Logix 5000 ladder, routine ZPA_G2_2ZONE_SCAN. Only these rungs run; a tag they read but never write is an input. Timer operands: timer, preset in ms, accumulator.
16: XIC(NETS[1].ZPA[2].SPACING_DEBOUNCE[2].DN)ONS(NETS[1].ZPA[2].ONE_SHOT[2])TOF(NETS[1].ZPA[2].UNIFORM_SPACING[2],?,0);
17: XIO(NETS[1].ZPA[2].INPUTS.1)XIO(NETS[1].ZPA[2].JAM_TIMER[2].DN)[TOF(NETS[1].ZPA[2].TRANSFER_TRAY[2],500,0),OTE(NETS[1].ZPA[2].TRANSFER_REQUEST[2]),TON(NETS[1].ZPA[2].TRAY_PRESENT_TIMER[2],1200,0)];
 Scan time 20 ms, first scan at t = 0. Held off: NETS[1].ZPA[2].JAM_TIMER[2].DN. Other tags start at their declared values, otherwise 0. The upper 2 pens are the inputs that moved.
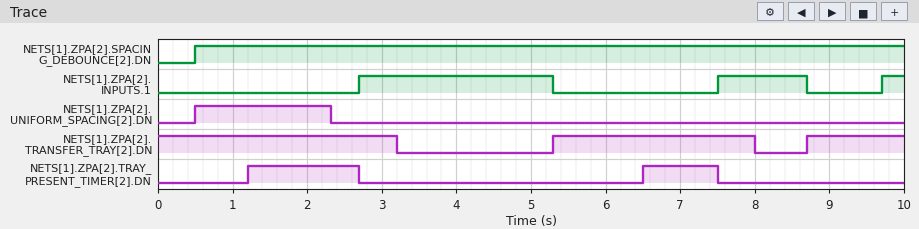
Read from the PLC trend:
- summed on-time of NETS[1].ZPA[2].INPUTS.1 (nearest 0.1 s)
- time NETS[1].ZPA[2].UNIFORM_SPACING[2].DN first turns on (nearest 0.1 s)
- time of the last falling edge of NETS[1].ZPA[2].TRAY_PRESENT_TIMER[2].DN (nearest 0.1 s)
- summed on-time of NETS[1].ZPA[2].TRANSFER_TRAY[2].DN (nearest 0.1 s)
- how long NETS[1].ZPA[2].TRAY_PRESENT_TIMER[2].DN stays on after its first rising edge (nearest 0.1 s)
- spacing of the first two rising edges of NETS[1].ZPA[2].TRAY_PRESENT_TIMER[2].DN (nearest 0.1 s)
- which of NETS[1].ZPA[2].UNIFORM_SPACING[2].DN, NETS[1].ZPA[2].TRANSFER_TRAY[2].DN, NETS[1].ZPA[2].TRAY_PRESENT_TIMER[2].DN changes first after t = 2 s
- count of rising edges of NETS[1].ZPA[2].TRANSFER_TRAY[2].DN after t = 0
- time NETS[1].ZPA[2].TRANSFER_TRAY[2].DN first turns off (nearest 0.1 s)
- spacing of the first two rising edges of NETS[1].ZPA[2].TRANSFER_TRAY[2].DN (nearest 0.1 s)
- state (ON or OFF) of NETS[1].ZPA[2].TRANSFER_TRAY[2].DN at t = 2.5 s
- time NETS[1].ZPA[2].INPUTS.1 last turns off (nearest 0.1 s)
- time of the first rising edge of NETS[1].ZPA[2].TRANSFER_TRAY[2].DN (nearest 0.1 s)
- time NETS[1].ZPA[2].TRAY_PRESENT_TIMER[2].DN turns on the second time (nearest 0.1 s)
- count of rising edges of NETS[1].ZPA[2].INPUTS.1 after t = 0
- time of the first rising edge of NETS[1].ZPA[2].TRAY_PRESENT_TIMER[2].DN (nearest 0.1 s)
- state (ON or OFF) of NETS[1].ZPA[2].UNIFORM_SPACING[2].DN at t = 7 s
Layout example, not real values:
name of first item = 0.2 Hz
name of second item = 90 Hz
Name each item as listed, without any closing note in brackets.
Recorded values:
summed on-time of NETS[1].ZPA[2].INPUTS.1 = 4.1 s
time NETS[1].ZPA[2].UNIFORM_SPACING[2].DN first turns on = 0.5 s
time of the last falling edge of NETS[1].ZPA[2].TRAY_PRESENT_TIMER[2].DN = 7.5 s
summed on-time of NETS[1].ZPA[2].TRANSFER_TRAY[2].DN = 7.2 s
how long NETS[1].ZPA[2].TRAY_PRESENT_TIMER[2].DN stays on after its first rising edge = 1.5 s
spacing of the first two rising edges of NETS[1].ZPA[2].TRAY_PRESENT_TIMER[2].DN = 5.3 s
which of NETS[1].ZPA[2].UNIFORM_SPACING[2].DN, NETS[1].ZPA[2].TRANSFER_TRAY[2].DN, NETS[1].ZPA[2].TRAY_PRESENT_TIMER[2].DN changes first after t = 2 s = NETS[1].ZPA[2].UNIFORM_SPACING[2].DN
count of rising edges of NETS[1].ZPA[2].TRANSFER_TRAY[2].DN after t = 0 = 2
time NETS[1].ZPA[2].TRANSFER_TRAY[2].DN first turns off = 3.2 s
spacing of the first two rising edges of NETS[1].ZPA[2].TRANSFER_TRAY[2].DN = 3.4 s
state (ON or OFF) of NETS[1].ZPA[2].TRANSFER_TRAY[2].DN at t = 2.5 s = ON
time NETS[1].ZPA[2].INPUTS.1 last turns off = 8.7 s
time of the first rising edge of NETS[1].ZPA[2].TRANSFER_TRAY[2].DN = 5.3 s
time NETS[1].ZPA[2].TRAY_PRESENT_TIMER[2].DN turns on the second time = 6.5 s
count of rising edges of NETS[1].ZPA[2].INPUTS.1 after t = 0 = 3
time of the first rising edge of NETS[1].ZPA[2].TRAY_PRESENT_TIMER[2].DN = 1.2 s
state (ON or OFF) of NETS[1].ZPA[2].UNIFORM_SPACING[2].DN at t = 7 s = OFF
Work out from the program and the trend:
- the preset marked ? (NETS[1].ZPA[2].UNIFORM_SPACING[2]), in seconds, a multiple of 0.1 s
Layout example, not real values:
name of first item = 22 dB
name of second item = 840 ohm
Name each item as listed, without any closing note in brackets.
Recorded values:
the preset marked ? (NETS[1].ZPA[2].UNIFORM_SPACING[2]), in seconds, a multiple of 0.1 s = 1.8 s
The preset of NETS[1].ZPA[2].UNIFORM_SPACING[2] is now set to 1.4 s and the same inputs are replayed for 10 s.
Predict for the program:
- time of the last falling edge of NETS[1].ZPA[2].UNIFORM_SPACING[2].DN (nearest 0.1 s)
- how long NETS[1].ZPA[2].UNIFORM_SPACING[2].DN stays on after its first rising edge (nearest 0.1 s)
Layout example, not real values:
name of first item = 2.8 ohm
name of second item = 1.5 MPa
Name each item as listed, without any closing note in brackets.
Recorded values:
time of the last falling edge of NETS[1].ZPA[2].UNIFORM_SPACING[2].DN = 1.9 s
how long NETS[1].ZPA[2].UNIFORM_SPACING[2].DN stays on after its first rising edge = 1.4 s
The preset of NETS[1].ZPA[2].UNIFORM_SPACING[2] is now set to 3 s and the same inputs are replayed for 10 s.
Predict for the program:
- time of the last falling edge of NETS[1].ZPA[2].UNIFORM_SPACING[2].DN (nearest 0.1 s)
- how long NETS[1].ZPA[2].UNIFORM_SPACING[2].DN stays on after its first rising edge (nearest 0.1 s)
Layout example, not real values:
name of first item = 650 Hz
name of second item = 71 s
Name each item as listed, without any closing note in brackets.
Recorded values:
time of the last falling edge of NETS[1].ZPA[2].UNIFORM_SPACING[2].DN = 3.5 s
how long NETS[1].ZPA[2].UNIFORM_SPACING[2].DN stays on after its first rising edge = 3.0 s
